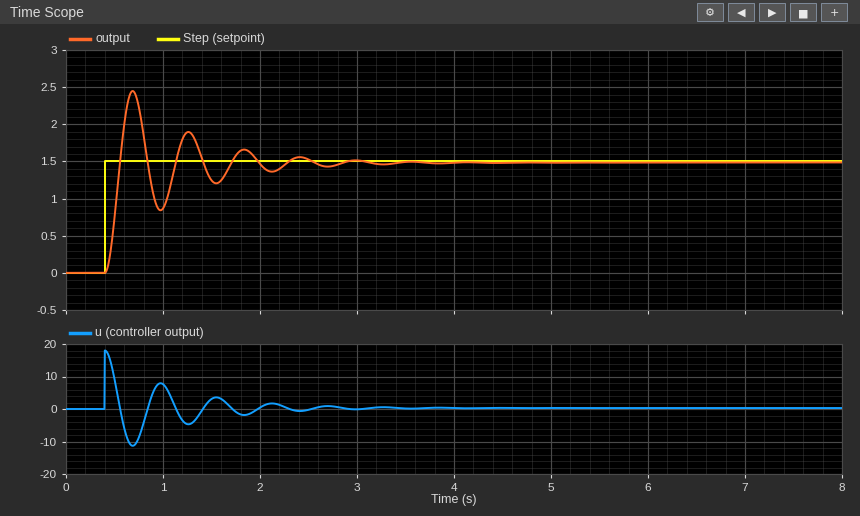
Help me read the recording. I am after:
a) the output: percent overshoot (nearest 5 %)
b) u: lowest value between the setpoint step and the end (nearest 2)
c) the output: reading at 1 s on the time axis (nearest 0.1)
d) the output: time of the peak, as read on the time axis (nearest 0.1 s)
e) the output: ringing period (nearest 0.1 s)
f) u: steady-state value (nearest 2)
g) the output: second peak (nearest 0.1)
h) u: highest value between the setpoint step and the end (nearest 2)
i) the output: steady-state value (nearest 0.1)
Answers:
65 %
-12
0.9
0.7 s
0.6 s
0
1.9
18
1.5
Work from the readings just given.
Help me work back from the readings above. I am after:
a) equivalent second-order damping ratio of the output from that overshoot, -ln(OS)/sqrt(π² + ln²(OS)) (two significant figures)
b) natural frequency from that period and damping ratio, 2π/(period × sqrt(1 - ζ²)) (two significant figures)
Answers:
0.14
11 rad/s
